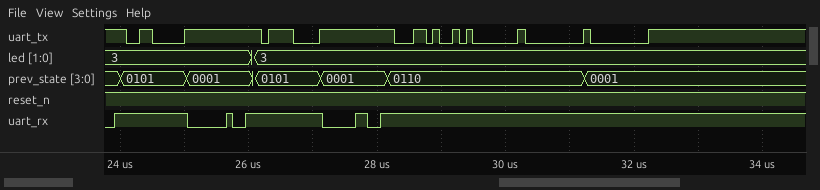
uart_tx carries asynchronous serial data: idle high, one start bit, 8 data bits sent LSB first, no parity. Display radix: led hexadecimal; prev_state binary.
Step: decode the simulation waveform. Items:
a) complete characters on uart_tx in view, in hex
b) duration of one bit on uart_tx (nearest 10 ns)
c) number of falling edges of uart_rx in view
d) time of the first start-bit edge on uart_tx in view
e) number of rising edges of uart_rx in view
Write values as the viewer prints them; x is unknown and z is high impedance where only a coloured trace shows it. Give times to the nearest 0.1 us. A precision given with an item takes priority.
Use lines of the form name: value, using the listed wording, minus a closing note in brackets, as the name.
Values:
complete characters on uart_tx in view, in hex: 06, 0F, 2C, 01, 00, 00
duration of one bit on uart_tx: 100 ns
number of falling edges of uart_rx in view: 4
time of the first start-bit edge on uart_tx in view: 24.1 us
number of rising edges of uart_rx in view: 5
